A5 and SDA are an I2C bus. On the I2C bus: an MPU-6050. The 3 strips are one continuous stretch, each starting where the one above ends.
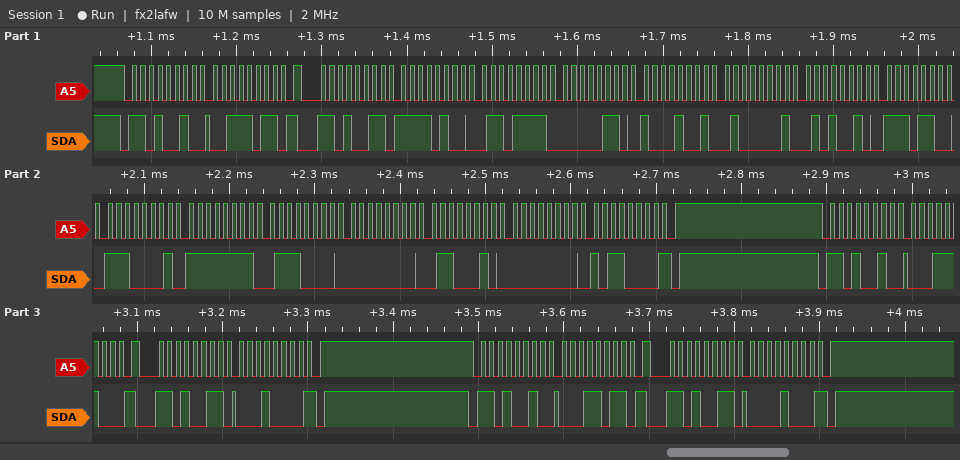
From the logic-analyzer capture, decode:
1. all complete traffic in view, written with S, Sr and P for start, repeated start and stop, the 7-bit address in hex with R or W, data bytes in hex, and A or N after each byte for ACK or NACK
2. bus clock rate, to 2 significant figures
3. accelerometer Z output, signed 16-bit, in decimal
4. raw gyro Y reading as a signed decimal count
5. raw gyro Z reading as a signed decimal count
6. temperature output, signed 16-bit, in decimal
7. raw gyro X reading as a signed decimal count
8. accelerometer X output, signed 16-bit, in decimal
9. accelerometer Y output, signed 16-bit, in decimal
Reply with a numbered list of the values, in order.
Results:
1. S 69W A 3B A Sr 69R A F4 A 6F A 06 A 89 A 41 A 52 A EC A E1 A FF A 70 A 00 A 62 A 00 A B0 N P S 69W A 1C A Sr 69R A 10 N P S 69W A 1B A Sr 69R A 08 N P
2. 100 kHz
3. 16722
4. 98
5. 176
6. -4895
7. -144
8. -2961
9. 1673
